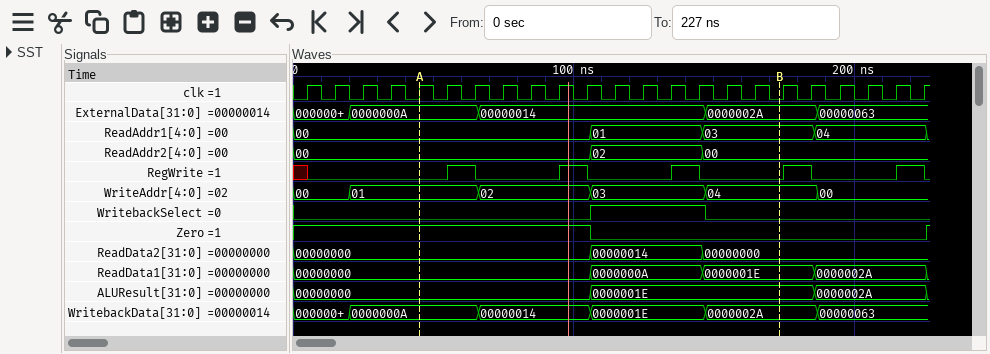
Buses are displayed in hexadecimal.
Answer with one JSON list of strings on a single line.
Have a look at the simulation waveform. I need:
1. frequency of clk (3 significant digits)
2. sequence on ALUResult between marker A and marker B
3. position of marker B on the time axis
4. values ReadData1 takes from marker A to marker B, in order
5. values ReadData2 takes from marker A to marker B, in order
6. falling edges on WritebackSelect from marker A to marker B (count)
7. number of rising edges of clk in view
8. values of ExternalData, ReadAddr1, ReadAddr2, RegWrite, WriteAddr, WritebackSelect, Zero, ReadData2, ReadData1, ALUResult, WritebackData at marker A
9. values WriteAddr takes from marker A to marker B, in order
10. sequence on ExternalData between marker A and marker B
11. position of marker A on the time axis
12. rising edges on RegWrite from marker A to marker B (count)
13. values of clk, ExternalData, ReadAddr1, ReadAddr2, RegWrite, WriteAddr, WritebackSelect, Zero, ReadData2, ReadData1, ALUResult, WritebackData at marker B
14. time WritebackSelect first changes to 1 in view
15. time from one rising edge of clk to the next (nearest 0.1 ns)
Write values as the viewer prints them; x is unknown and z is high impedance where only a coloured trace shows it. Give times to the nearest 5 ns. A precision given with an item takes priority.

["100 MHz", "00000000, 0000001E", "175 ns", "00000000, 0000000A, 0000001E", "00000000, 00000014, 00000000", "1", "23", "ExternalData=0000000A, ReadAddr1=00, ReadAddr2=00, RegWrite=0, WriteAddr=01, WritebackSelect=0, Zero=1, ReadData2=00000000, ReadData1=00000000, ALUResult=00000000, WritebackData=0000000A", "01, 02, 03, 04", "0000000A, 00000014, 0000002A", "45 ns", "3", "clk=0, ExternalData=0000002A, ReadAddr1=03, ReadAddr2=00, RegWrite=0, WriteAddr=04, WritebackSelect=0, Zero=0, ReadData2=00000000, ReadData1=0000001E, ALUResult=0000001E, WritebackData=0000002A", "105 ns", "10 ns"]
